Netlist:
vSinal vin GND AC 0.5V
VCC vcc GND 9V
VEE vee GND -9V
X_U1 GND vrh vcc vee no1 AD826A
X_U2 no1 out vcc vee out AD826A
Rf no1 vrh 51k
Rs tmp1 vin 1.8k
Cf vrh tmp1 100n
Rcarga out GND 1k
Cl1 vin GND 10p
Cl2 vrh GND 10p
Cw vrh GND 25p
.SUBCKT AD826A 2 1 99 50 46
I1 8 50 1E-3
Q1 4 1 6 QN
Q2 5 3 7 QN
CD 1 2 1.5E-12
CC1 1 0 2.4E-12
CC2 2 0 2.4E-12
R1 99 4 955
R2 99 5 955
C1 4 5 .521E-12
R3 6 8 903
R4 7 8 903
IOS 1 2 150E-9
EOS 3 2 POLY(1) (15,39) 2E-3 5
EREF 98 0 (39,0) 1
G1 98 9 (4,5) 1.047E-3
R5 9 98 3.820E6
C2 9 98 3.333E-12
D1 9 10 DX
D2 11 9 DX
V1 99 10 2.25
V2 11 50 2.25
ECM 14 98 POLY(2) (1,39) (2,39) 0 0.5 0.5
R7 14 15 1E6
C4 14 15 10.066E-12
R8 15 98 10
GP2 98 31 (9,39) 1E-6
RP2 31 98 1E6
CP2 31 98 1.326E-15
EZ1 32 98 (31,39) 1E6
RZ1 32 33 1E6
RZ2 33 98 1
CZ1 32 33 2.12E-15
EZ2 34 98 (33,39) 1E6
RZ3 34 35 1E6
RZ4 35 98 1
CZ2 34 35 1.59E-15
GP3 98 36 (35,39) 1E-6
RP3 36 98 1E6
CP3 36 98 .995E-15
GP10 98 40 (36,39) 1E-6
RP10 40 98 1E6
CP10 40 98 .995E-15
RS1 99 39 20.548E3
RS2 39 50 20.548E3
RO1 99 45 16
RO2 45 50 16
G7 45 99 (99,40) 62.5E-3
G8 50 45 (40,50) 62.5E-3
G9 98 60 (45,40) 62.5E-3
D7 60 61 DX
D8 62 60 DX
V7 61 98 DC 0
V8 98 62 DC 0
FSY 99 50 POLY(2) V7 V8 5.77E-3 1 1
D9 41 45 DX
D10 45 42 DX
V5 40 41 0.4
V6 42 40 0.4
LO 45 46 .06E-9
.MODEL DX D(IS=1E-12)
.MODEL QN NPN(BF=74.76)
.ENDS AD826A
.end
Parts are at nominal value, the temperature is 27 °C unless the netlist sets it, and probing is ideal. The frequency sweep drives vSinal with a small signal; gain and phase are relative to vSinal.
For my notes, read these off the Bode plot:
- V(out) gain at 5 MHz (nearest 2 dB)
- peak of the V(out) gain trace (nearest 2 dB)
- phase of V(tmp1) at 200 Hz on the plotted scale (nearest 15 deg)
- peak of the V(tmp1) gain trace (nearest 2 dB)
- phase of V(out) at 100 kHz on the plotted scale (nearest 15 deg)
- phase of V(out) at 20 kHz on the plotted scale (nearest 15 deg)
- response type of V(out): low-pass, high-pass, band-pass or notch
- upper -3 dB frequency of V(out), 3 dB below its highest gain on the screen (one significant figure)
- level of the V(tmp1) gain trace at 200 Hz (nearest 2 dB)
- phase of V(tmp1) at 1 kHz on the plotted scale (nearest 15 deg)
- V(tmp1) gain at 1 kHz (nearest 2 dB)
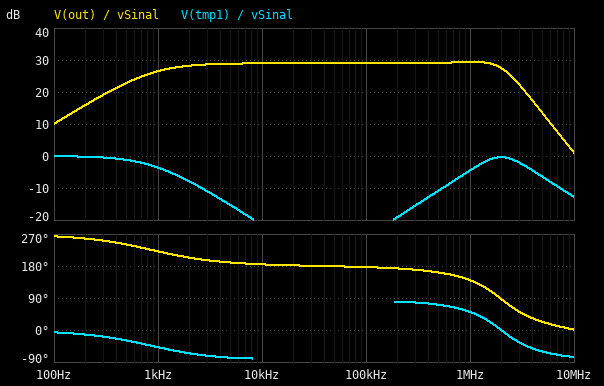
14 dB
30 dB
-15 deg
0 dB
180 deg
180 deg
band-pass
2 MHz
0 dB
-45 deg
-4 dB
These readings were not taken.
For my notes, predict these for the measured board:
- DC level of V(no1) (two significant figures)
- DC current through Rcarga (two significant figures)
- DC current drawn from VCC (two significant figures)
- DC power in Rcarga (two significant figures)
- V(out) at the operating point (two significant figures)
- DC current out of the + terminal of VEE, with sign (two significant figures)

350 mV
350 µA
15 mA
120 µW
350 mV
-14 mA
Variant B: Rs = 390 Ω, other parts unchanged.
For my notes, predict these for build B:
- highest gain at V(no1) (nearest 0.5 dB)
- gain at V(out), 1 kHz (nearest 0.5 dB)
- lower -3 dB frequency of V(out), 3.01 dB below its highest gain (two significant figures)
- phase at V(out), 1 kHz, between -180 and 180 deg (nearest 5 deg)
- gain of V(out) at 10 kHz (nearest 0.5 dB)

42.0 dB
30.0 dB
3.9 kHz
-105 deg
41.5 dB
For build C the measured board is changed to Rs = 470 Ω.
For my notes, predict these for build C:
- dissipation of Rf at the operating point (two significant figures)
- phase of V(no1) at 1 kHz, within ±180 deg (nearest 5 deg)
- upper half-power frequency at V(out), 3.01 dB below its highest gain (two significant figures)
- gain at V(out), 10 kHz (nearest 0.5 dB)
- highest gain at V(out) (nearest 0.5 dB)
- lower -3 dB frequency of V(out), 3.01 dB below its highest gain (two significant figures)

2.3 µW
-105 deg
490 kHz
40.0 dB
40.5 dB
3.3 kHz
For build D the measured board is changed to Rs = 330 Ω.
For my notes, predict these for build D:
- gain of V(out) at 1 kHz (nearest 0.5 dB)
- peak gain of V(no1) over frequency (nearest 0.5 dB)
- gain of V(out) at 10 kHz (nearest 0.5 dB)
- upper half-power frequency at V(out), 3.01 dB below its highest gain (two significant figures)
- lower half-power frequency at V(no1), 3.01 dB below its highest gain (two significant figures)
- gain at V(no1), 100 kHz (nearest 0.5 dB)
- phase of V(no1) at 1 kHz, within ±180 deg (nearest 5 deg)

30.0 dB
43.5 dB
42.5 dB
340 kHz
4.6 kHz
43.0 dB
-100 deg
